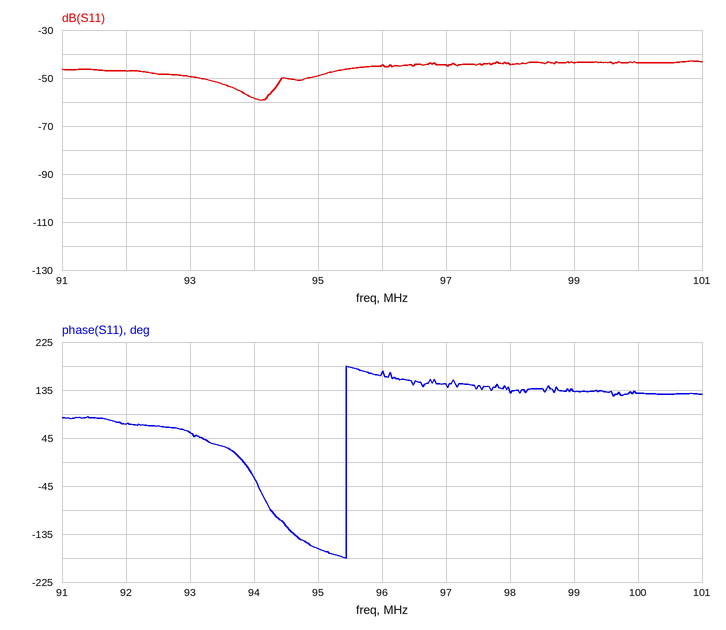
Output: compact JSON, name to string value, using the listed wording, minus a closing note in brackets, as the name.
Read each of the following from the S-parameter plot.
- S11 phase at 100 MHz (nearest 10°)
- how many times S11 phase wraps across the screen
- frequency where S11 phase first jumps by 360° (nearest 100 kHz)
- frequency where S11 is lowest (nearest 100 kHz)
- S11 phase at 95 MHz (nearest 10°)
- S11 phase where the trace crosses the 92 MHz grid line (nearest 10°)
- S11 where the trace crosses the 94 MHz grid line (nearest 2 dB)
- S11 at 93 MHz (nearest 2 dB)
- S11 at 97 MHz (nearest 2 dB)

{"S11 phase at 100 MHz": "130°", "how many times S11 phase wraps across the screen": "1", "frequency where S11 phase first jumps by 360°": "95.4 MHz", "frequency where S11 is lowest": "94.1 MHz", "S11 phase at 95 MHz": "-160°", "S11 phase where the trace crosses the 92 MHz grid line": "70°", "S11 where the trace crosses the 94 MHz grid line": "-58 dB", "S11 at 93 MHz": "-50 dB", "S11 at 97 MHz": "-44 dB"}
